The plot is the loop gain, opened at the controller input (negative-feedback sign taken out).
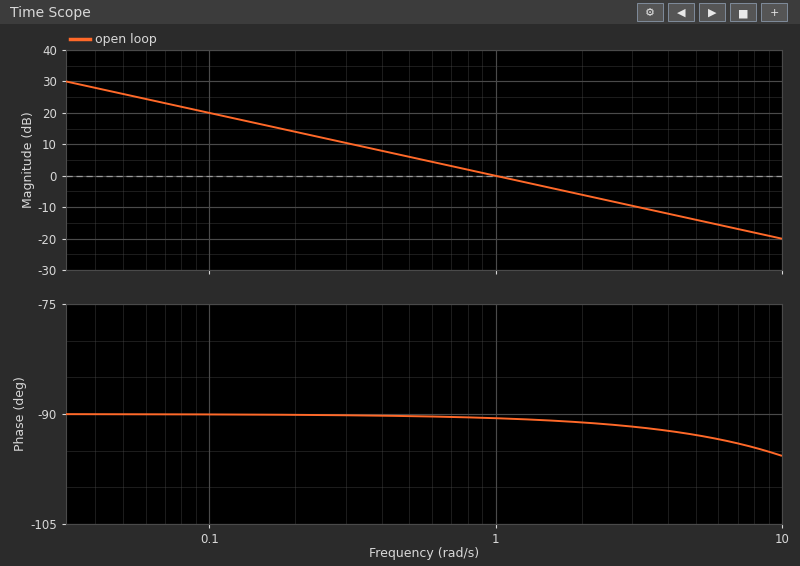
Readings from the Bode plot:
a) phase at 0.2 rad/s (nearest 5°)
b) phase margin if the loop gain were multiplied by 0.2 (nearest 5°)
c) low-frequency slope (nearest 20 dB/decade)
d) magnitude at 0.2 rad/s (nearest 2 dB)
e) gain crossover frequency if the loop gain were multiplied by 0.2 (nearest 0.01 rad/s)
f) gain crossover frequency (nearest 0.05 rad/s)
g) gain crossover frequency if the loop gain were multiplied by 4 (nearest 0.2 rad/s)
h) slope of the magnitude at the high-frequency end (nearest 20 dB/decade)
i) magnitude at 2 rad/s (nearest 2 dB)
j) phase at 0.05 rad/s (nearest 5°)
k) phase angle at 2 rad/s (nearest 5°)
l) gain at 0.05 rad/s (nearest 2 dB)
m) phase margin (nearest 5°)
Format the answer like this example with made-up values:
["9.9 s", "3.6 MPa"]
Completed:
["-90°", "90°", "-20 dB/decade", "14 dB", "0.20 rad/s", "1.00 rad/s", "4.0 rad/s", "-20 dB/decade", "-6 dB", "-90°", "-90°", "26 dB", "90°"]
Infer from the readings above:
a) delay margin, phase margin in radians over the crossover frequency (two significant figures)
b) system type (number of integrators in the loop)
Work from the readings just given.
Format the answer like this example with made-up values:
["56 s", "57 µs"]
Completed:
["1.6 s", "1"]
